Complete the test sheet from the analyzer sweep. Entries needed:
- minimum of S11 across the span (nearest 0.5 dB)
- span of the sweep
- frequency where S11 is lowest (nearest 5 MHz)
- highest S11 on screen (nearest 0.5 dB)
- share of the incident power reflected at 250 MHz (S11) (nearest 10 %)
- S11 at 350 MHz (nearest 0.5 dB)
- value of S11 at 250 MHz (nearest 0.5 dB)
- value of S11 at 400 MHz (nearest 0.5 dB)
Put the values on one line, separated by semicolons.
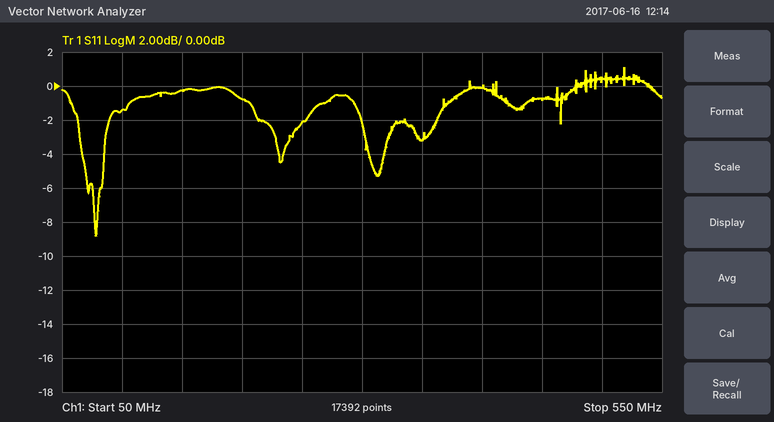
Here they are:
-9.0 dB; 500 MHz; 80 MHz; 1.0 dB; 60 %; -3.0 dB; -2.0 dB; 0.0 dB
